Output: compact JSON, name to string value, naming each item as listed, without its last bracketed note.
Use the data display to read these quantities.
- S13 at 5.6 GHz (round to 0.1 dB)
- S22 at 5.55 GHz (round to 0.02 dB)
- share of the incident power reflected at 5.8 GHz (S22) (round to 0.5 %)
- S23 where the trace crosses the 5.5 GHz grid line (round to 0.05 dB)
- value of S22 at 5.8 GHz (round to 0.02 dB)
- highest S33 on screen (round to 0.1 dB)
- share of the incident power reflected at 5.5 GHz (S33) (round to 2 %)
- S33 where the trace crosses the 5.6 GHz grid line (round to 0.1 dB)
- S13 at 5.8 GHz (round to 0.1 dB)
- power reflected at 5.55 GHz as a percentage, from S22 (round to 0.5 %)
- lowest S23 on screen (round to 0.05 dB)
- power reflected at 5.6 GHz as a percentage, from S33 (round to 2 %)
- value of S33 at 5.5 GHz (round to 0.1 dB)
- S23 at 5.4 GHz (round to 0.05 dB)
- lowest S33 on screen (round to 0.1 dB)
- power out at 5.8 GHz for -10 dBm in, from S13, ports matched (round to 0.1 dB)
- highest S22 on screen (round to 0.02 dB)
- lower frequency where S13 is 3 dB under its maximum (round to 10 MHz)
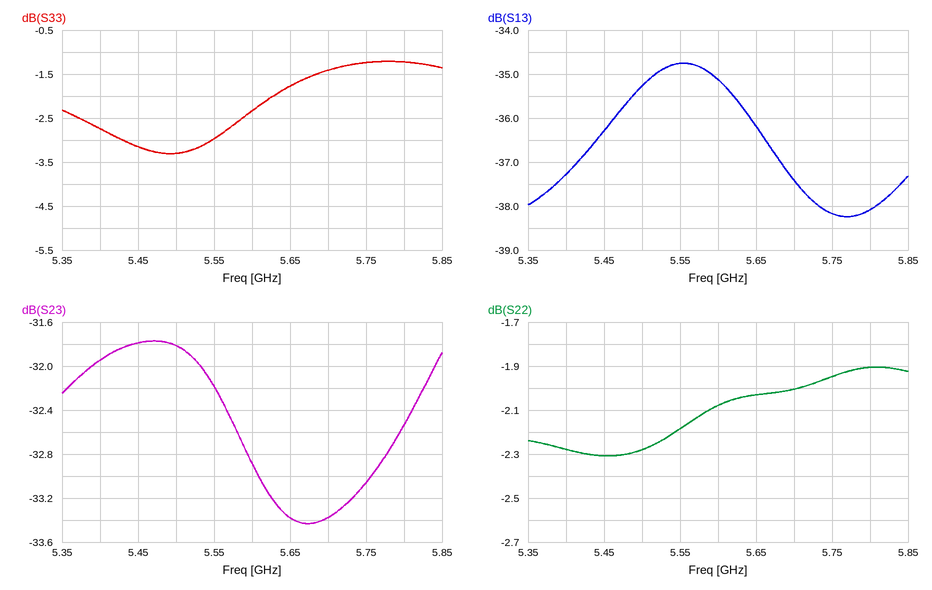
{"S13 at 5.6 GHz": "-35.1 dB", "S22 at 5.55 GHz": "-2.18 dB", "share of the incident power reflected at 5.8 GHz (S22)": "64.5 %", "S23 where the trace crosses the 5.5 GHz grid line": "-31.80 dB", "value of S22 at 5.8 GHz": "-1.90 dB", "highest S33 on screen": "-1.2 dB", "share of the incident power reflected at 5.5 GHz (S33)": "46 %", "S33 where the trace crosses the 5.6 GHz grid line": "-2.3 dB", "S13 at 5.8 GHz": "-38.1 dB", "power reflected at 5.55 GHz as a percentage, from S22": "60.5 %", "lowest S23 on screen": "-33.45 dB", "power reflected at 5.6 GHz as a percentage, from S33": "58 %", "value of S33 at 5.5 GHz": "-3.3 dB", "S23 at 5.4 GHz": "-31.95 dB", "lowest S33 on screen": "-3.3 dB", "power out at 5.8 GHz for -10 dBm in, from S13, ports matched": "-48.1 dBm", "highest S22 on screen": "-1.90 dB", "lower frequency where S13 is 3 dB under its maximum": "5.37 GHz"}
